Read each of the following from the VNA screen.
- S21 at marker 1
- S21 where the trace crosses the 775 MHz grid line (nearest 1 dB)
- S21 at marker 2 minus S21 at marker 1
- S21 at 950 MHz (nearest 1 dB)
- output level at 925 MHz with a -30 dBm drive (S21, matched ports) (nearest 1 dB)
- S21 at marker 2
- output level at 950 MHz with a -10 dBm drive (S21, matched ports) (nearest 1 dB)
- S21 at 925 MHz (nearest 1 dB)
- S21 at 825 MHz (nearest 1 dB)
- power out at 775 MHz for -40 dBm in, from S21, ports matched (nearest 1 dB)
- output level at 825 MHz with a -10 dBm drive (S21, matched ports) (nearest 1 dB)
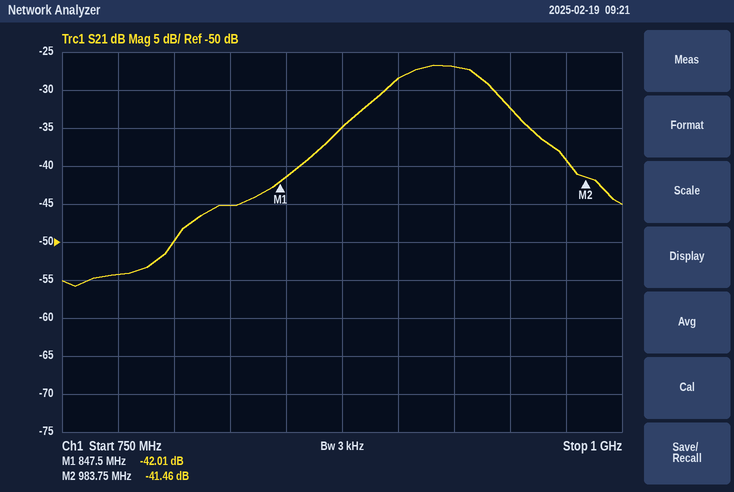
-42.01 dB
-54 dB
0.55 dB
-32 dB
-57 dBm
-41.46 dB
-42 dBm
-27 dB
-45 dB
-94 dBm
-55 dBm
